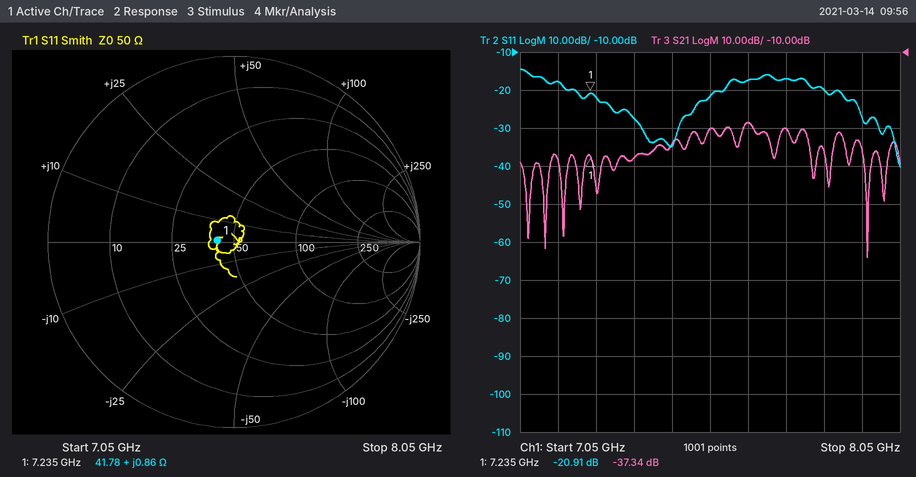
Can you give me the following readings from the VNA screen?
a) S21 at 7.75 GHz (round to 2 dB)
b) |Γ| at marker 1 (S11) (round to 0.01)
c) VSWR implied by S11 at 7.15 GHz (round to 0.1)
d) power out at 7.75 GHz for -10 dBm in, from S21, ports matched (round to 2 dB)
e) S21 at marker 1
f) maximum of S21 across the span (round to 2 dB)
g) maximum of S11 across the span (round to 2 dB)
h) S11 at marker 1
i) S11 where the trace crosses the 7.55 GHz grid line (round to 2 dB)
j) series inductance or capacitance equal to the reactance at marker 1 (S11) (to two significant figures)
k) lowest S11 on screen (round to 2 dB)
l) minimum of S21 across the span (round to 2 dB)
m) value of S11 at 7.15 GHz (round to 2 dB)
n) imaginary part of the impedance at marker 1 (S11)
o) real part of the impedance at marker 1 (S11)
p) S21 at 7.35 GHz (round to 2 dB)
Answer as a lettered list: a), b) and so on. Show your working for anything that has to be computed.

a) -30 dB
b) 0.09
c) |Γ| = 10^(-18/20) = 0.1259; VSWR = (1 + 0.1259)/(1 − 0.1259) ≈ 1.3
d) -10 dBm + (-30 dB) = -40 dBm
e) -37.34 dB
f) -28 dB
g) -14 dB
h) -20.91 dB
i) -22 dB
j) L = 0.86 Ω/(2π × 7.235 GHz) ≈ 19 pH
k) -40 dB
l) -64 dB
m) -18 dB
n) +0.86 Ω
o) 41.78 Ω
p) -38 dB
